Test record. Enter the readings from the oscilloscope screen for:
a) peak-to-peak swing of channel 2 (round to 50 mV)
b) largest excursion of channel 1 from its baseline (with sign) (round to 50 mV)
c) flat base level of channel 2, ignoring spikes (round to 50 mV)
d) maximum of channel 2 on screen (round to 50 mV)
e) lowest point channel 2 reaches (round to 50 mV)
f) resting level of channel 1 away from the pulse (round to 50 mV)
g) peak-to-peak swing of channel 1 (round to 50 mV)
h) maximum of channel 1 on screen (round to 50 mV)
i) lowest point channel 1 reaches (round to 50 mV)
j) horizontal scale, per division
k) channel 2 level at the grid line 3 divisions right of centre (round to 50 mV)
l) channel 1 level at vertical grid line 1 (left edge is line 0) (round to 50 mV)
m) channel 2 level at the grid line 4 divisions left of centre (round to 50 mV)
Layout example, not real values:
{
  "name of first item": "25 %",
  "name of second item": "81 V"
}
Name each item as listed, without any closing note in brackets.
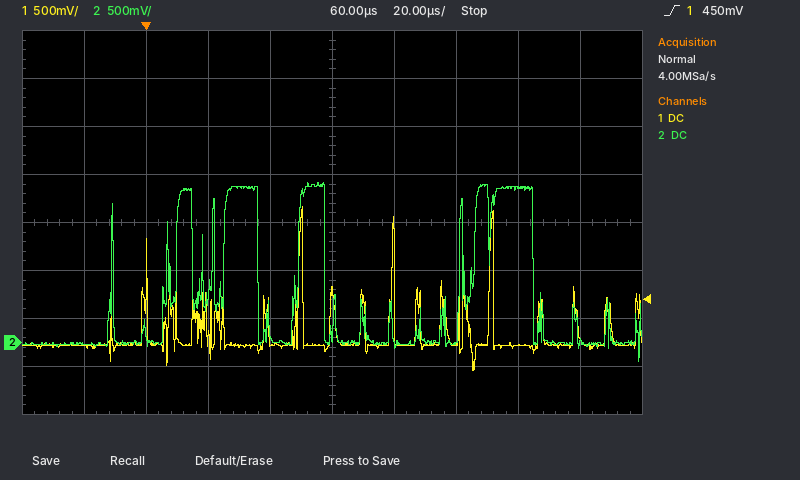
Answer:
{
  "peak-to-peak swing of channel 2": "1.85 V",
  "largest excursion of channel 1 from its baseline (with sign)": "+1.45 V",
  "flat base level of channel 2, ignoring spikes": "0 mV",
  "maximum of channel 2 on screen": "1.65 V",
  "lowest point channel 2 reaches": "-200 mV",
  "resting level of channel 1 away from the pulse": "-50 mV",
  "peak-to-peak swing of channel 1": "1.70 V",
  "maximum of channel 1 on screen": "1.40 V",
  "lowest point channel 1 reaches": "-300 mV",
  "horizontal scale, per division": "20 µs",
  "channel 2 level at the grid line 3 divisions right of centre": "1.60 V",
  "channel 1 level at vertical grid line 1 (left edge is line 0)": "-50 mV",
  "channel 2 level at the grid line 4 divisions left of centre": "0 mV"
}
